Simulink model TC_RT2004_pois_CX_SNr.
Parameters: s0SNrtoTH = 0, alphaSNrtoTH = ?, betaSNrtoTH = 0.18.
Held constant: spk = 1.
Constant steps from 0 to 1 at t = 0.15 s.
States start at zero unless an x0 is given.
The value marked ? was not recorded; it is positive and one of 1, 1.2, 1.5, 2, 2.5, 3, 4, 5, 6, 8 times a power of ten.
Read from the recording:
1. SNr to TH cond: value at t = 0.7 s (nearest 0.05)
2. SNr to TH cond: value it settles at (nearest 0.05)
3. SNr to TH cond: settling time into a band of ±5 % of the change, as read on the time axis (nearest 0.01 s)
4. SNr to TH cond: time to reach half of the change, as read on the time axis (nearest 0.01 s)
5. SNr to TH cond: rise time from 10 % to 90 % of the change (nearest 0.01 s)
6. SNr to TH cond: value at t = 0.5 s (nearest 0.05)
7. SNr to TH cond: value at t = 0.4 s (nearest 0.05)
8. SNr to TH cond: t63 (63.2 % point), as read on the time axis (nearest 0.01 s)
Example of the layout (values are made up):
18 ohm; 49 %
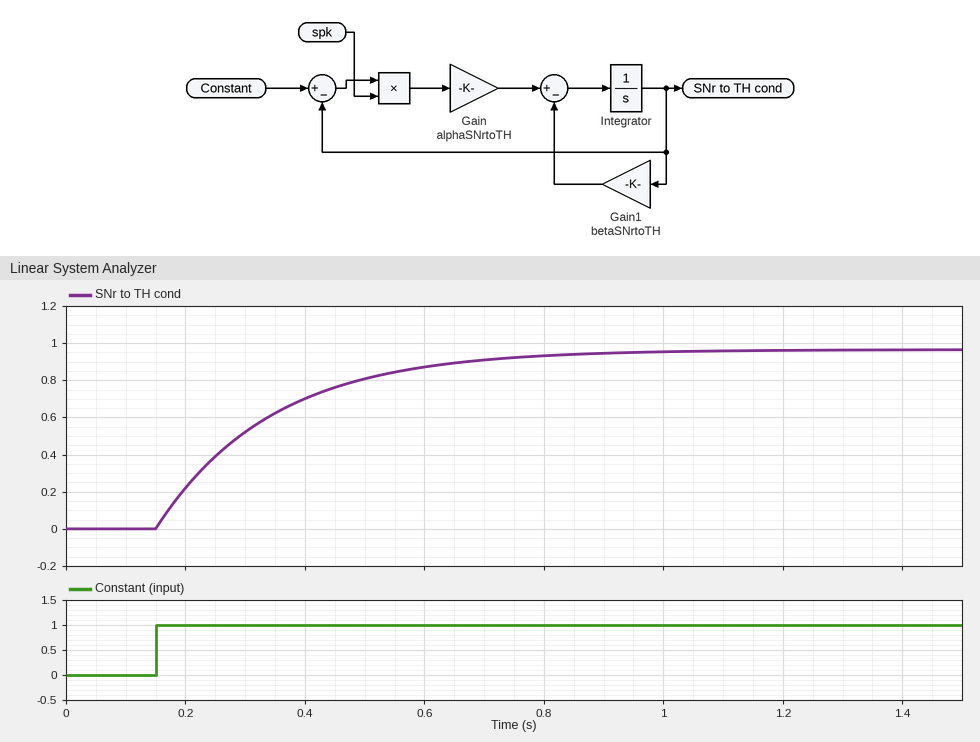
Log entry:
0.90; 0.95; 0.73 s; 0.28 s; 0.42 s; 0.80; 0.70; 0.34 s
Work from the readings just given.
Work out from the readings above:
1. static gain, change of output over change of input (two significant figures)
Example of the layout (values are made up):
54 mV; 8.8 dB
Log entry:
0.95
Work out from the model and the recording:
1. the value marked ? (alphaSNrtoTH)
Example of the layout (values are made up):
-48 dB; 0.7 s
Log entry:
5
